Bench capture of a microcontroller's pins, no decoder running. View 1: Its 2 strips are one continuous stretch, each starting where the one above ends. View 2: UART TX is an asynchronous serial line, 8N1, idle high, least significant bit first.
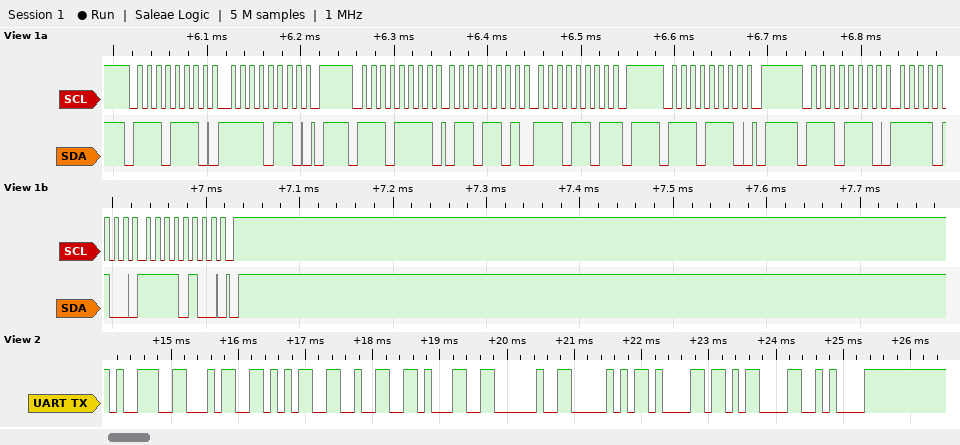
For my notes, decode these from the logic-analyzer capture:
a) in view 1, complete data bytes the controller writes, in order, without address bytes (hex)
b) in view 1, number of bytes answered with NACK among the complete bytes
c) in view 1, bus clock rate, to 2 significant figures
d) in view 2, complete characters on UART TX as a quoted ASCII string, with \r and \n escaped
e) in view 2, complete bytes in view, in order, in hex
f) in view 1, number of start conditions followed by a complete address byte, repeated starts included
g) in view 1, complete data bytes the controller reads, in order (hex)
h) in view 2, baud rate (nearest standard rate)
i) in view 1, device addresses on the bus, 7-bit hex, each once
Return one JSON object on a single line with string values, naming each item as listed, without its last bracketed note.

{"in view 1, complete data bytes the controller writes, in order, without address bytes": "F6 F4 F4", "in view 1, number of bytes answered with NACK among the complete bytes": "1", "in view 1, bus clock rate, to 2 significant figures": "100 kHz", "in view 2, complete characters on UART TX as a quoted ASCII string, with \\r and \\n escaped": "\"94521 Pa\\r\\n\"", "in view 2, complete bytes in view, in order, in hex": "39 34 35 32 31 20 50 61 0D 0A", "in view 1, number of start conditions followed by a complete address byte, repeated starts included": "4", "in view 1, complete data bytes the controller reads, in order": "6D ED", "in view 2, baud rate": "9600 baud", "in view 1, device addresses on the bus, 7-bit hex, each once": "0x77"}
